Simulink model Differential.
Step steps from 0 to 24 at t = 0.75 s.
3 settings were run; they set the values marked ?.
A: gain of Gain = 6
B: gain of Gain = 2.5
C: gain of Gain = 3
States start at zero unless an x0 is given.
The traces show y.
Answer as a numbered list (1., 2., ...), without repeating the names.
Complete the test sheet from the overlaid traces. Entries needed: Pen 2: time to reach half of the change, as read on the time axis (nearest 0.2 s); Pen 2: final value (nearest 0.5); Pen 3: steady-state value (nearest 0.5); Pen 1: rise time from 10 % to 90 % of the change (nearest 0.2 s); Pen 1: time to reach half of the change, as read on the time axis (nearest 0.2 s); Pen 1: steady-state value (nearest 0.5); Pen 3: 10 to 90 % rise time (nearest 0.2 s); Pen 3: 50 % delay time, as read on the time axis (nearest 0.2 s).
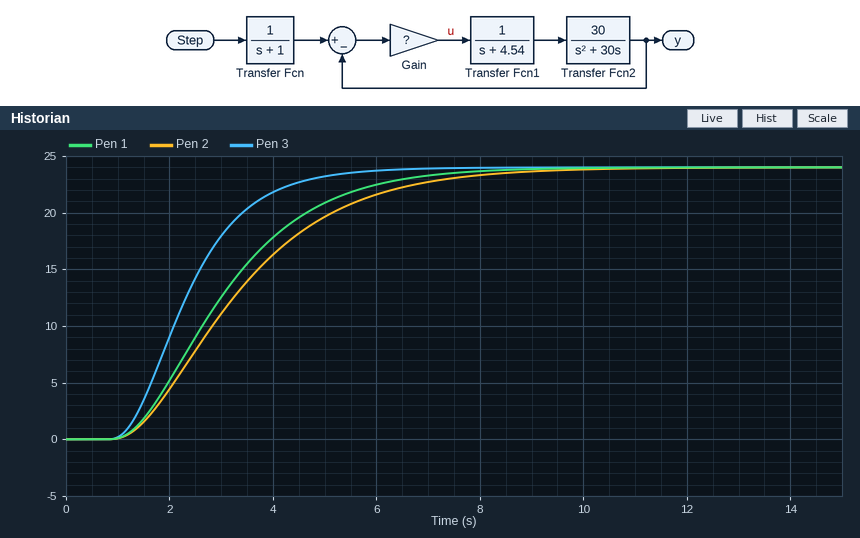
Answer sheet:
1. 3.2 s
2. 24.0
3. 24.0
4. 3.8 s
5. 3.0 s
6. 24.0
7. 2.6 s
8. 2.2 s
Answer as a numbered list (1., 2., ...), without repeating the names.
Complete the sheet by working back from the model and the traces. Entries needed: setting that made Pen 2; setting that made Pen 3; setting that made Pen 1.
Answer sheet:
1. B
2. A
3. C
